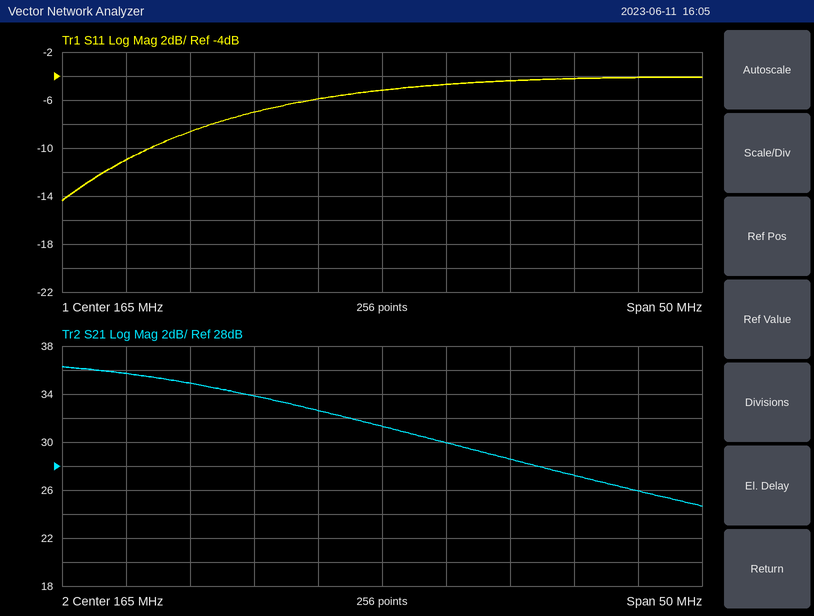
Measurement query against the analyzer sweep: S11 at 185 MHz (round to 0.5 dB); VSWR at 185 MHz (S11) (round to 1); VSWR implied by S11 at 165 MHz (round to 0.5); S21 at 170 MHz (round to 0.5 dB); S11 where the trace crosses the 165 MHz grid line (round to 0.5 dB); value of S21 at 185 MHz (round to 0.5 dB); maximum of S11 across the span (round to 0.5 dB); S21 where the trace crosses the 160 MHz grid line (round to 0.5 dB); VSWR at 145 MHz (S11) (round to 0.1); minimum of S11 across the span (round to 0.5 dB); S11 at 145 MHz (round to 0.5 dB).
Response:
-4.0 dB
4
3.5
30.0 dB
-5.0 dB
26.0 dB
-4.0 dB
32.5 dB
1.8
-14.5 dB
-11.0 dB
